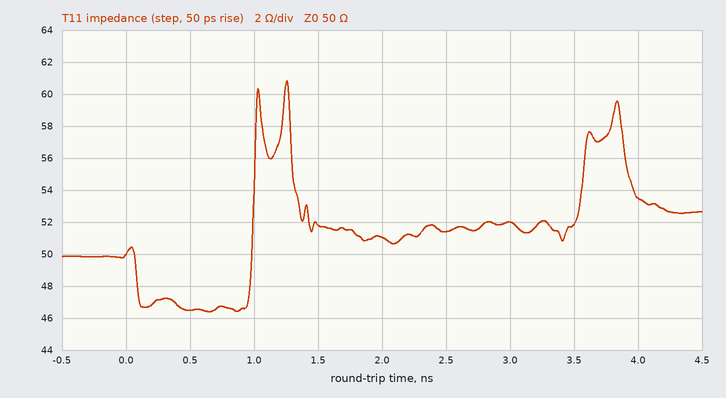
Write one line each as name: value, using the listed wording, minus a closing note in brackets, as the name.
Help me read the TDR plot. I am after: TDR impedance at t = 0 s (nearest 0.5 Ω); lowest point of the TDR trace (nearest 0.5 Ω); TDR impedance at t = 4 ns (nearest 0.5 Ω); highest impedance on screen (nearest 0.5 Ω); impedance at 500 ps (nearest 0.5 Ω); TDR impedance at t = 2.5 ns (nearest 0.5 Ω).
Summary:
TDR impedance at t = 0 s: 50.0 Ω
lowest point of the TDR trace: 46.5 Ω
TDR impedance at t = 4 ns: 53.5 Ω
highest impedance on screen: 61.0 Ω
impedance at 500 ps: 46.5 Ω
TDR impedance at t = 2.5 ns: 51.5 Ω
